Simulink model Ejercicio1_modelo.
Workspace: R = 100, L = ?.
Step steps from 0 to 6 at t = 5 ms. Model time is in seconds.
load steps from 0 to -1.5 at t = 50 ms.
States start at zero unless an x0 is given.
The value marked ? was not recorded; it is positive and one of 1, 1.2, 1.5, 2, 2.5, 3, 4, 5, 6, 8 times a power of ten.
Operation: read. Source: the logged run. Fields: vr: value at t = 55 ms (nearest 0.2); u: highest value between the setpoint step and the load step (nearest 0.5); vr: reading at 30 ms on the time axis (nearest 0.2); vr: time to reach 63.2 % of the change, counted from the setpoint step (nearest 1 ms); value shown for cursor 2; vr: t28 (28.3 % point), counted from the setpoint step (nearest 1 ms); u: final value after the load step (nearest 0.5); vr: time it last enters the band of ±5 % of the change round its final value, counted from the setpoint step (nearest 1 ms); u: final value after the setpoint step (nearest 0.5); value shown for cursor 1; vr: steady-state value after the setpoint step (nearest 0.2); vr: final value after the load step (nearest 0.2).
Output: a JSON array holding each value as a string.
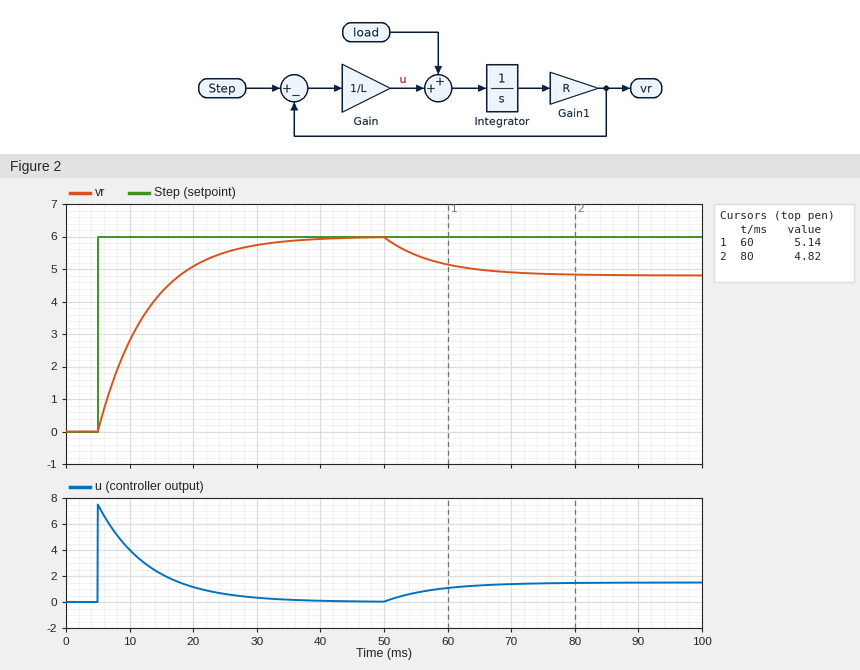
["5.4", "7.5", "5.8", "8 ms", "4.82", "3 ms", "1.5", "24 ms", "0.0", "5.14", "6.0", "4.8"]
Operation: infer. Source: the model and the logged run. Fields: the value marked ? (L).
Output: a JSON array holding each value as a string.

["0.8"]
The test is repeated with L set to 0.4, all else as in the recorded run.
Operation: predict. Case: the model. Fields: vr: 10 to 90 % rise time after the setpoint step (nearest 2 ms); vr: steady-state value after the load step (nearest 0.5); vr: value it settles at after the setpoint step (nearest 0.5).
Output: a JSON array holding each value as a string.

["8 ms", "5.5", "6.0"]
